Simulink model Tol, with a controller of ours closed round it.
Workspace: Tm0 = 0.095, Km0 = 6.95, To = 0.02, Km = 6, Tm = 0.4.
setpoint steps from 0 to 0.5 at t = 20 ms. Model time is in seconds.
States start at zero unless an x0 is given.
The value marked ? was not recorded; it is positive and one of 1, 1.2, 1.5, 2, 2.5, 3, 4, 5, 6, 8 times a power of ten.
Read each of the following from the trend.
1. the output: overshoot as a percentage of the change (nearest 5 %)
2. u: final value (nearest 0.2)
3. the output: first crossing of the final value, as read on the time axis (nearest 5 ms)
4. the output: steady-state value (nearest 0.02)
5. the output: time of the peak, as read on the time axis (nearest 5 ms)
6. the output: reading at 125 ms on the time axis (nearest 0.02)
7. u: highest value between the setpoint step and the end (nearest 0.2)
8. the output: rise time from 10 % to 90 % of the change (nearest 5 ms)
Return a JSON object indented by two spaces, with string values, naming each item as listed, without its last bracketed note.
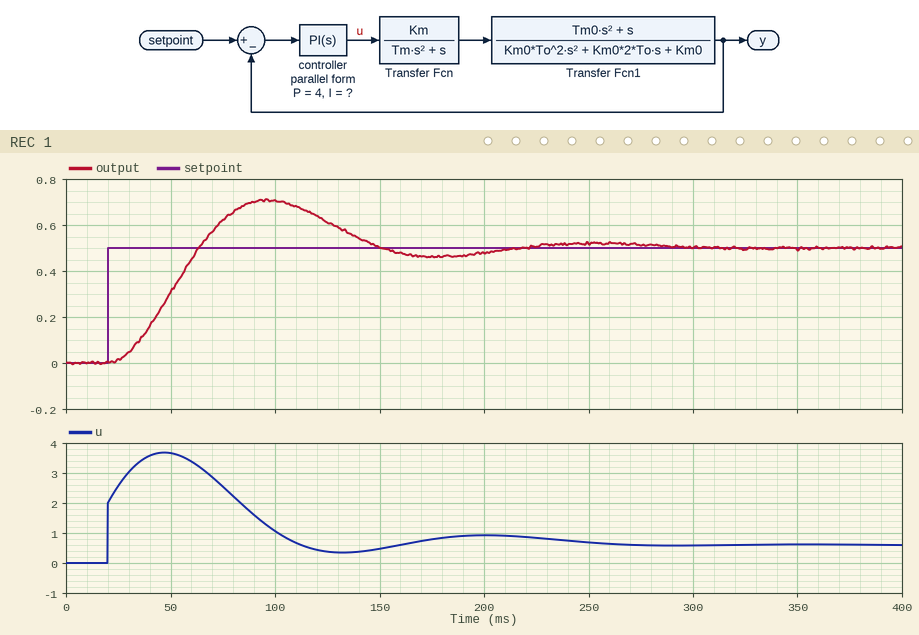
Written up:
{
  "the output: overshoot as a percentage of the change": "40 %",
  "u: final value": "0.6",
  "the output: first crossing of the final value, as read on the time axis": "65 ms",
  "the output: steady-state value": "0.50",
  "the output: time of the peak, as read on the time axis": "95 ms",
  "the output: reading at 125 ms on the time axis": "0.62",
  "u: highest value between the setpoint step and the end": "3.6",
  "the output: rise time from 10 % to 90 % of the change": "30 ms"
}
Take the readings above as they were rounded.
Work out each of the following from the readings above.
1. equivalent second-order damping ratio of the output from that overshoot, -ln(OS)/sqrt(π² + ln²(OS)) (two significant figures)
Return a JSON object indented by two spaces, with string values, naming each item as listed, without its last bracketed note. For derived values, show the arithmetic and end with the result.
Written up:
{
  "equivalent second-order damping ratio of the output from that overshoot, -ln(OS)/sqrt(π² + ln²(OS))": "ln(0.4) = -0.916; 0.916 / sqrt(9.870 + 0.840) = 0.28"
}
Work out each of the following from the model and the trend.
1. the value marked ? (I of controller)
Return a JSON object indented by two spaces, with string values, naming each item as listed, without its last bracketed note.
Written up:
{
  "the value marked ?": "250"
}
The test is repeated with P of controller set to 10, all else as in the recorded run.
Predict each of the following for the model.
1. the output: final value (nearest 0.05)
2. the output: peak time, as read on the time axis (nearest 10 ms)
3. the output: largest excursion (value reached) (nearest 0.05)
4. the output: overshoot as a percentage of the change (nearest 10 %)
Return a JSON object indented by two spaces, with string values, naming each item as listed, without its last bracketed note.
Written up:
{
  "the output: final value": "0.50",
  "the output: peak time, as read on the time axis": "70 ms",
  "the output: largest excursion (value reached)": "0.60",
  "the output: overshoot as a percentage of the change": "20 %"
}
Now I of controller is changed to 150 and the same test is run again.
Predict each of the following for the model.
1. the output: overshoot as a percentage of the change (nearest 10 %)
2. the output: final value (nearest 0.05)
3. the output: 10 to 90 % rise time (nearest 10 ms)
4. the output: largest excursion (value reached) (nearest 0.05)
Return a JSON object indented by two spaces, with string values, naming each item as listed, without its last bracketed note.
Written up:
{
  "the output: overshoot as a percentage of the change": "20 %",
  "the output: final value": "0.50",
  "the output: 10 to 90 % rise time": "40 ms",
  "the output: largest excursion (value reached)": "0.60"
}
